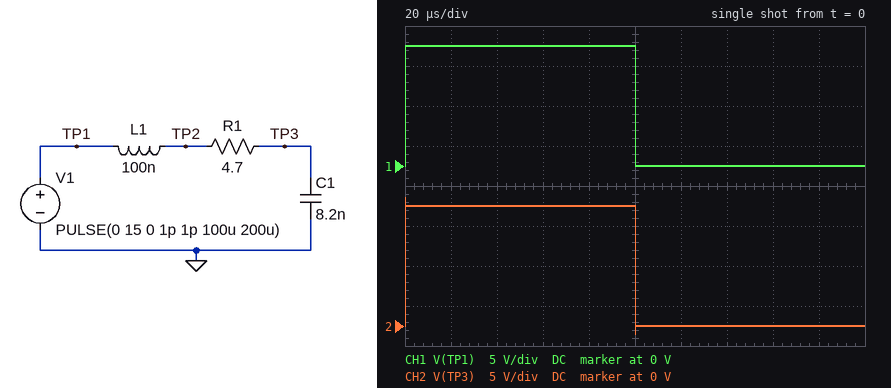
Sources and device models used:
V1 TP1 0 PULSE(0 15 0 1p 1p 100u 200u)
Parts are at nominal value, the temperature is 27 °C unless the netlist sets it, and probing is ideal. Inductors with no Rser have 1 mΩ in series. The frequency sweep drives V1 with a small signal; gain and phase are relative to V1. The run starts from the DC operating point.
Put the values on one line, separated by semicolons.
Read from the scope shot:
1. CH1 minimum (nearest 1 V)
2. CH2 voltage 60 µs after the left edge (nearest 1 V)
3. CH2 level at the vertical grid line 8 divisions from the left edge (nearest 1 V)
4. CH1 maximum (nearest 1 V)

0 V; 15 V; 0 V; 15 V
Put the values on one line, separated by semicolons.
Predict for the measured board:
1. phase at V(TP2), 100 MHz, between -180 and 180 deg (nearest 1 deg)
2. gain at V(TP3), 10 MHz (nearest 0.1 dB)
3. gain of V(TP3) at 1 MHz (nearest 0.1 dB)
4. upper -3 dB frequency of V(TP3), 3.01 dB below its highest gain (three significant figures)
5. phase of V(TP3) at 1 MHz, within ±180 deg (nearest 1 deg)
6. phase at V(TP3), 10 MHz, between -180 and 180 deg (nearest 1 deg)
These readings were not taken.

-88 deg; -10.4 dB; 0 dB; 5.80 MHz; -14 deg; -133 deg
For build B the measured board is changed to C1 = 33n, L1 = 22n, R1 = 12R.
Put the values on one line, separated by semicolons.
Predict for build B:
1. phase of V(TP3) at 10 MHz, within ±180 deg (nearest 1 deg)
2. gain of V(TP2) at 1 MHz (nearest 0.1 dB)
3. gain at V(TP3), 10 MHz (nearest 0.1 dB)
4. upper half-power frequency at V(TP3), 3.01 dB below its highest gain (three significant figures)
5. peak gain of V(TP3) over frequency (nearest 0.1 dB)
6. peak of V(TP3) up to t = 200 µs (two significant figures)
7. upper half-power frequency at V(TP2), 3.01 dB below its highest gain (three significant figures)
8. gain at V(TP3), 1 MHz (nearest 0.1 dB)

-94 deg; 0 dB; -27.9 dB; 404 kHz; 0 dB; 15 V; 86.5 MHz; -8.5 dB
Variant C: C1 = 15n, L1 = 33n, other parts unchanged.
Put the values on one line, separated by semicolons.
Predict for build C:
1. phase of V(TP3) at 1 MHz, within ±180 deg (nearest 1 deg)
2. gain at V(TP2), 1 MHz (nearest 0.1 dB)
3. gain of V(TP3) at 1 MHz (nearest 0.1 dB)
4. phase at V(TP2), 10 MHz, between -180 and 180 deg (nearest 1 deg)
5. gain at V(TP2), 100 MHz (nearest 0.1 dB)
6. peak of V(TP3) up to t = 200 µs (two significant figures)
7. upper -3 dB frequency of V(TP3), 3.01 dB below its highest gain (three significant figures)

-24 deg; 0.1 dB; -0.6 dB; -25 deg; -13.1 dB; 15 V; 2.50 MHz
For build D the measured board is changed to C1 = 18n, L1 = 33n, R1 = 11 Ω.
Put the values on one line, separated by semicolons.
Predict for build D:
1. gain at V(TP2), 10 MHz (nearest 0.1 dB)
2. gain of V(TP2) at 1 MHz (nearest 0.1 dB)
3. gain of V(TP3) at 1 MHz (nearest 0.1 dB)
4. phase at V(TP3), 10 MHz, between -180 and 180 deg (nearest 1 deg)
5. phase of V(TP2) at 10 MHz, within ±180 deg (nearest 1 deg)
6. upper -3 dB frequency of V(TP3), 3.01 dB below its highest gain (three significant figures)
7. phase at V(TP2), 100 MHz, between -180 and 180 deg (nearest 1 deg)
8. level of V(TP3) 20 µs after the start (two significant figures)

0 dB; 0.1 dB; -4.0 dB; -96 deg; -11 deg; 816 kHz; -62 deg; 15 V
